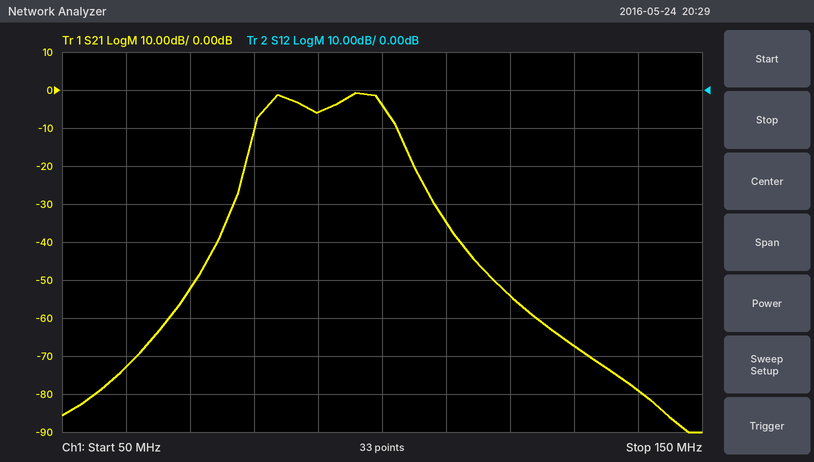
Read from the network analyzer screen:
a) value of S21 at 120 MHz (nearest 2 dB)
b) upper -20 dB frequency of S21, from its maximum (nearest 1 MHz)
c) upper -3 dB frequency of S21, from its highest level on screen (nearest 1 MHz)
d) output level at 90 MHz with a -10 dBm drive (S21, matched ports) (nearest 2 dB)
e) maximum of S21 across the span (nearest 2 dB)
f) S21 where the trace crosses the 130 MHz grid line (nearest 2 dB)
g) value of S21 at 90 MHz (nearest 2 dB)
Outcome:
-54 dB
105 MHz
100 MHz
-16 dBm
0 dB
-68 dB
-6 dB
